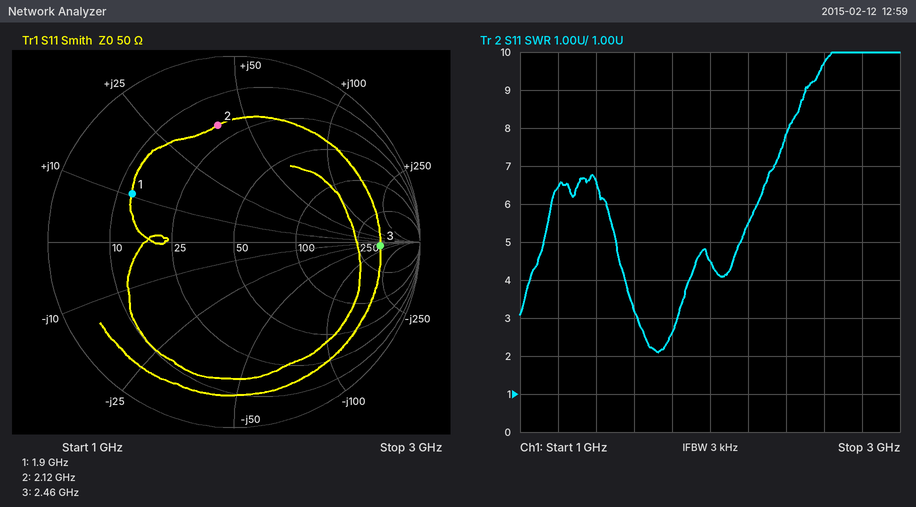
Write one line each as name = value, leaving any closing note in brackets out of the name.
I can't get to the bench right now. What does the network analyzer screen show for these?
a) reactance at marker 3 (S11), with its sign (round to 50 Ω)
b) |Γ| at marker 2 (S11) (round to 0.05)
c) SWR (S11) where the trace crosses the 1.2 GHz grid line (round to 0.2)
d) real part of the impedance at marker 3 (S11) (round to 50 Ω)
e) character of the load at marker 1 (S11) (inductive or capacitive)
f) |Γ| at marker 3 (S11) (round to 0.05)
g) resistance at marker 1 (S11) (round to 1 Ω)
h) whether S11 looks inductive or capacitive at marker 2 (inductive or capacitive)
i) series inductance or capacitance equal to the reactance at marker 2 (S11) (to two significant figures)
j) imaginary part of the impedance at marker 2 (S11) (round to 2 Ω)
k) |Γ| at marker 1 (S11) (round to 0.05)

reactance at marker 3 (S11), with its sign = -50 Ω
|Γ| at marker 2 (S11) = 0.65
SWR (S11) where the trace crosses the 1.2 GHz grid line = 6.4
real part of the impedance at marker 3 (S11) = 400 Ω
character of the load at marker 1 (S11) = inductive
|Γ| at marker 3 (S11) = 0.80
resistance at marker 1 (S11) = 13 Ω
whether S11 looks inductive or capacitive at marker 2 = inductive
series inductance or capacitance equal to the reactance at marker 2 (S11) = 3.0 nH
imaginary part of the impedance at marker 2 (S11) = +40 Ω
|Γ| at marker 1 (S11) = 0.60
